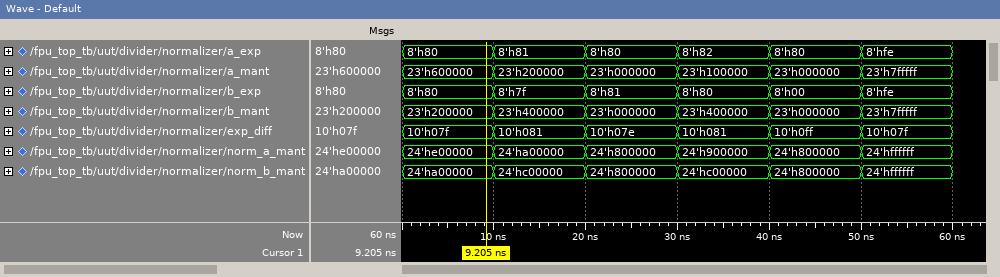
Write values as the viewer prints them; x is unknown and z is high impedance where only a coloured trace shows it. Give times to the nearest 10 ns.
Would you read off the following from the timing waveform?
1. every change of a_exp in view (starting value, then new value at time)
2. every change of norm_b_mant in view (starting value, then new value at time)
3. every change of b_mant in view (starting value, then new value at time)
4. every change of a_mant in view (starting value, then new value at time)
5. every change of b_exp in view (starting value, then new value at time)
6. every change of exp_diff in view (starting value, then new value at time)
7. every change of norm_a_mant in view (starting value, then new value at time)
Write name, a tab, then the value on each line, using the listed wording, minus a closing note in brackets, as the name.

every change of a_exp in view	8'h80, 8'h81 at 10 ns, 8'h80 at 20 ns, 8'h82 at 30 ns, 8'h80 at 40 ns, 8'hfe at 50 ns
every change of norm_b_mant in view	24'ha00000, 24'hc00000 at 10 ns, 24'h800000 at 20 ns, 24'hc00000 at 30 ns, 24'h800000 at 40 ns, 24'hffffff at 50 ns
every change of b_mant in view	23'h200000, 23'h400000 at 10 ns, 23'h000000 at 20 ns, 23'h400000 at 30 ns, 23'h000000 at 40 ns, 23'h7fffff at 50 ns
every change of a_mant in view	23'h600000, 23'h200000 at 10 ns, 23'h000000 at 20 ns, 23'h100000 at 30 ns, 23'h000000 at 40 ns, 23'h7fffff at 50 ns
every change of b_exp in view	8'h80, 8'h7f at 10 ns, 8'h81 at 20 ns, 8'h80 at 30 ns, 8'h00 at 40 ns, 8'hfe at 50 ns
every change of exp_diff in view	10'h07f, 10'h081 at 10 ns, 10'h07e at 20 ns, 10'h081 at 30 ns, 10'h0ff at 40 ns, 10'h07f at 50 ns
every change of norm_a_mant in view	24'he00000, 24'ha00000 at 10 ns, 24'h800000 at 20 ns, 24'h900000 at 30 ns, 24'h800000 at 40 ns, 24'hffffff at 50 ns
